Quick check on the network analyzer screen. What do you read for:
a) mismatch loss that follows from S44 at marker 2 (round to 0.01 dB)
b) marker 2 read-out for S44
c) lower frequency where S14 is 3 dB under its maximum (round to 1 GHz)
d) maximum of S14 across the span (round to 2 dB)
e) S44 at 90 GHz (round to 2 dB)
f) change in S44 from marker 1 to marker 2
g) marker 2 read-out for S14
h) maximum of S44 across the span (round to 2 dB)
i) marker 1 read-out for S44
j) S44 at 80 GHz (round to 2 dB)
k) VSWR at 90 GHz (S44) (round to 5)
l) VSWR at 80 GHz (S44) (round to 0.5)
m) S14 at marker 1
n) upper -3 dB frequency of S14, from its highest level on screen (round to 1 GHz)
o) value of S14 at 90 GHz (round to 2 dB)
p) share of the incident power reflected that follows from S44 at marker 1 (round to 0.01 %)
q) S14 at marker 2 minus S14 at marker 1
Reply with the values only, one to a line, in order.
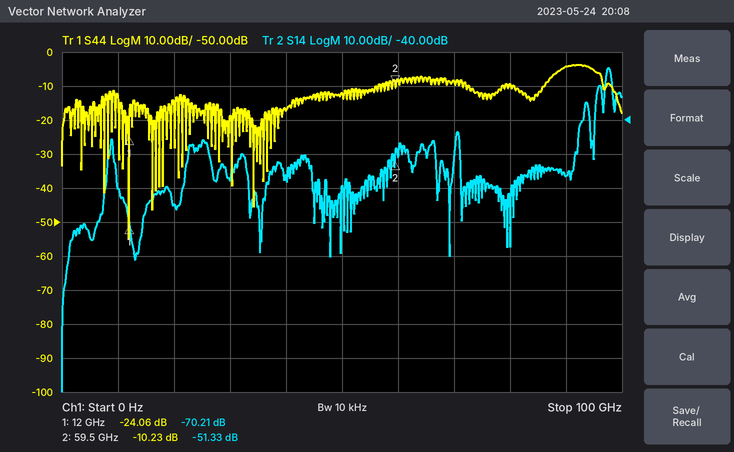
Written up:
0.43 dB
-10.23 dB
97 GHz
-24 dB
-4 dB
13.83 dB
-51.33 dB
-4 dB
-24.06 dB
-10 dB
5
2.0
-70.21 dB
98 GHz
-56 dB
0.39 %
18.88 dB
